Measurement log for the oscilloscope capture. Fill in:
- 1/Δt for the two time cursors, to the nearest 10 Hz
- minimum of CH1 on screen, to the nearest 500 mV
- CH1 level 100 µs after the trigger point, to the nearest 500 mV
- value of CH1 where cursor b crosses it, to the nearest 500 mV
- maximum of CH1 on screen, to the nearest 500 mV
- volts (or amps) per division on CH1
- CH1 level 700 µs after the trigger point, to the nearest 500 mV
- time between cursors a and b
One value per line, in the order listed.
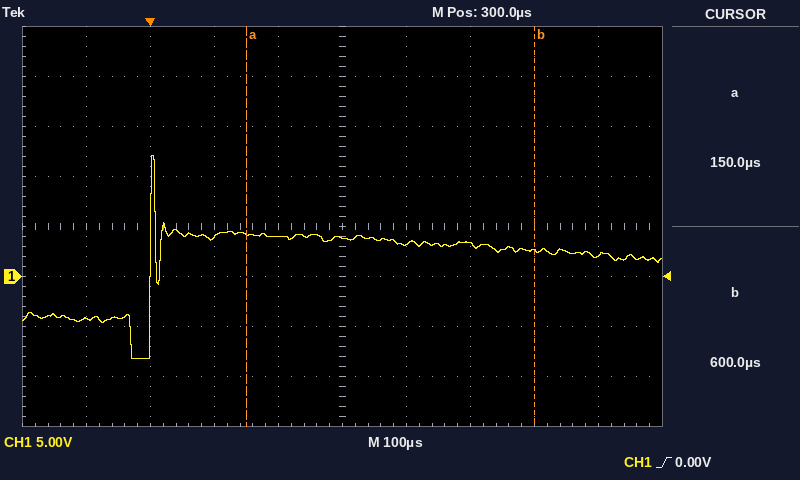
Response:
2.22 kHz
-8.0 V
4.0 V
2.5 V
12.0 V
5 V
2.0 V
450 µs
